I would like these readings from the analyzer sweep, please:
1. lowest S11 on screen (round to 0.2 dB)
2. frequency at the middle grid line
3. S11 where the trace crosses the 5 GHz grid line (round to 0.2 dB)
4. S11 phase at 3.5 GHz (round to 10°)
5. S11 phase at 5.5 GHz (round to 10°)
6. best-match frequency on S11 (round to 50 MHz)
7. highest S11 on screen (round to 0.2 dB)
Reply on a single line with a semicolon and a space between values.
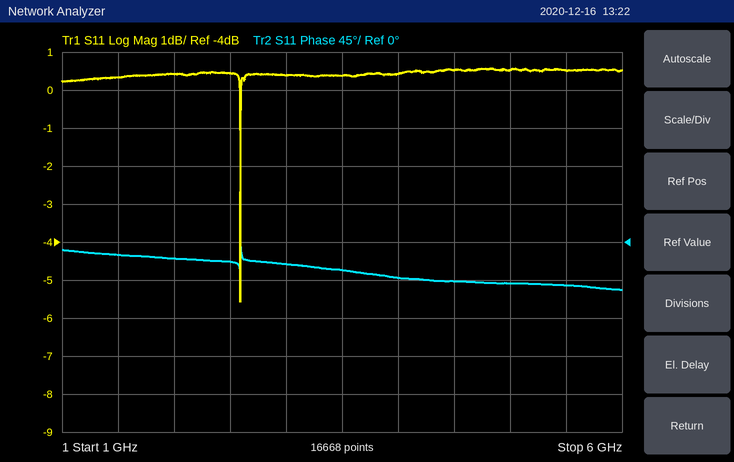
-5.6 dB; 3.5 GHz; 0.6 dB; -30°; -50°; 2.60 GHz; 0.6 dB
